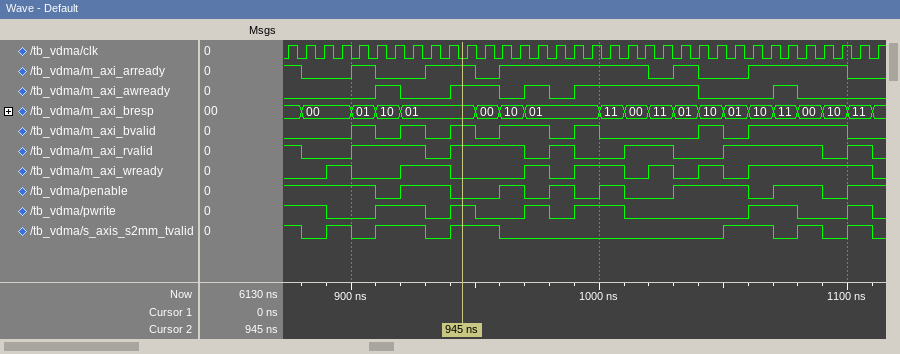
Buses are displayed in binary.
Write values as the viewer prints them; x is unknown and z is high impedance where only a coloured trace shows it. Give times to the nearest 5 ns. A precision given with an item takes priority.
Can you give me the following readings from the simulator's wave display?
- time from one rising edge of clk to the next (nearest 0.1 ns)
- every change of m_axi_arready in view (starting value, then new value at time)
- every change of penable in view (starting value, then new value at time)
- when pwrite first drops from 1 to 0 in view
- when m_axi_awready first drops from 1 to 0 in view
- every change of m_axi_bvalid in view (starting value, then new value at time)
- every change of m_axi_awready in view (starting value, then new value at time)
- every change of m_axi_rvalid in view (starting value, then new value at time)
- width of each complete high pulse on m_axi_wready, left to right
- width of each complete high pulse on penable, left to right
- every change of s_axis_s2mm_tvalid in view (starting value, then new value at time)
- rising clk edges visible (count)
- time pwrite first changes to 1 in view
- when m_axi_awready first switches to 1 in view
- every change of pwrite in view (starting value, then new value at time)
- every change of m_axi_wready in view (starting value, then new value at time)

7.2 ns
1, 0 at 880 ns, 1 at 900 ns, 0 at 910 ns, 1 at 930 ns, 0 at 950 ns, 1 at 960 ns, 0 at 1020 ns, 1 at 1030 ns, 0 at 1040 ns, 1 at 1060 ns, 0 at 1100 ns
1, 0 at 910 ns, 1 at 920 ns, 0 at 940 ns, 1 at 960 ns, 0 at 970 ns, 1 at 980 ns, 0 at 990 ns, 1 at 1000 ns, 0 at 1010 ns, 1 at 1030 ns, 0 at 1060 ns, 1 at 1070 ns, 0 at 1090 ns, 1 at 1100 ns
890 ns
920 ns
0, 1 at 900 ns, 0 at 910 ns, 1 at 920 ns, 0 at 930 ns, 1 at 940 ns, 0 at 950 ns, 1 at 960 ns, 0 at 980 ns, 1 at 990 ns, 0 at 1000 ns, 1 at 1040 ns, 0 at 1050 ns, 1 at 1060 ns, 0 at 1100 ns
0, 1 at 910 ns, 0 at 920 ns, 1 at 940 ns, 0 at 960 ns, 1 at 970 ns, 0 at 980 ns, 1 at 990 ns, 0 at 1040 ns, 1 at 1070 ns, 0 at 1080 ns
1, 0 at 880 ns, 1 at 900 ns, 0 at 930 ns, 1 at 940 ns, 0 at 970 ns, 1 at 980 ns, 0 at 990 ns, 1 at 1010 ns, 0 at 1030 ns, 1 at 1050 ns, 0 at 1090 ns, 1 at 1100 ns, 0 at 1110 ns
10 ns, 20 ns, 10 ns, 20 ns, 10 ns, 10 ns, 50 ns
20 ns, 10 ns, 10 ns, 10 ns, 30 ns, 20 ns
1, 0 at 880 ns, 1 at 890 ns, 0 at 900 ns, 1 at 910 ns, 0 at 930 ns, 1 at 940 ns, 0 at 960 ns, 1 at 1050 ns, 0 at 1070 ns, 1 at 1080 ns, 0 at 1090 ns, 1 at 1100 ns, 0 at 1110 ns
34
910 ns
910 ns
1, 0 at 890 ns, 1 at 910 ns, 0 at 930 ns, 1 at 940 ns, 0 at 950 ns, 1 at 970 ns, 0 at 980 ns, 1 at 990 ns, 0 at 1010 ns, 1 at 1060 ns, 0 at 1080 ns, 1 at 1100 ns, 0 at 1110 ns
0, 1 at 890 ns, 0 at 900 ns, 1 at 920 ns, 0 at 940 ns, 1 at 970 ns, 0 at 980 ns, 1 at 990 ns, 0 at 1010 ns, 1 at 1020 ns, 0 at 1030 ns, 1 at 1040 ns, 0 at 1050 ns, 1 at 1060 ns, 0 at 1110 ns
